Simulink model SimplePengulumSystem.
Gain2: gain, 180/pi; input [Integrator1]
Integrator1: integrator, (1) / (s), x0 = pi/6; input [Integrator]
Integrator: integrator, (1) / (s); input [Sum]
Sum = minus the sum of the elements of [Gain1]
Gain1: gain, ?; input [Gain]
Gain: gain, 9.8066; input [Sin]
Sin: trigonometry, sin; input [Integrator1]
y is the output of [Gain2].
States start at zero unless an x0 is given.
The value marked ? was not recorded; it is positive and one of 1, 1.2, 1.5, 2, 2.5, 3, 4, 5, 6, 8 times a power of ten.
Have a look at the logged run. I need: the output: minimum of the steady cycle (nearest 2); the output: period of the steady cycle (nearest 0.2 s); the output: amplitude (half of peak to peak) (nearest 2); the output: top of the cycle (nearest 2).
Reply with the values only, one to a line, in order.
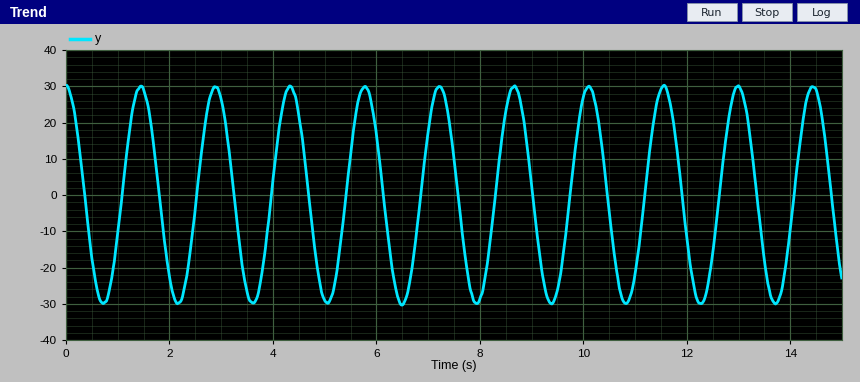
-30
1.4 s
30
30
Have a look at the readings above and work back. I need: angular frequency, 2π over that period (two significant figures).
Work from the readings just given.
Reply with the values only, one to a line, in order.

4.5 rad/s
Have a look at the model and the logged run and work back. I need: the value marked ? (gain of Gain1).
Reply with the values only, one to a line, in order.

2
